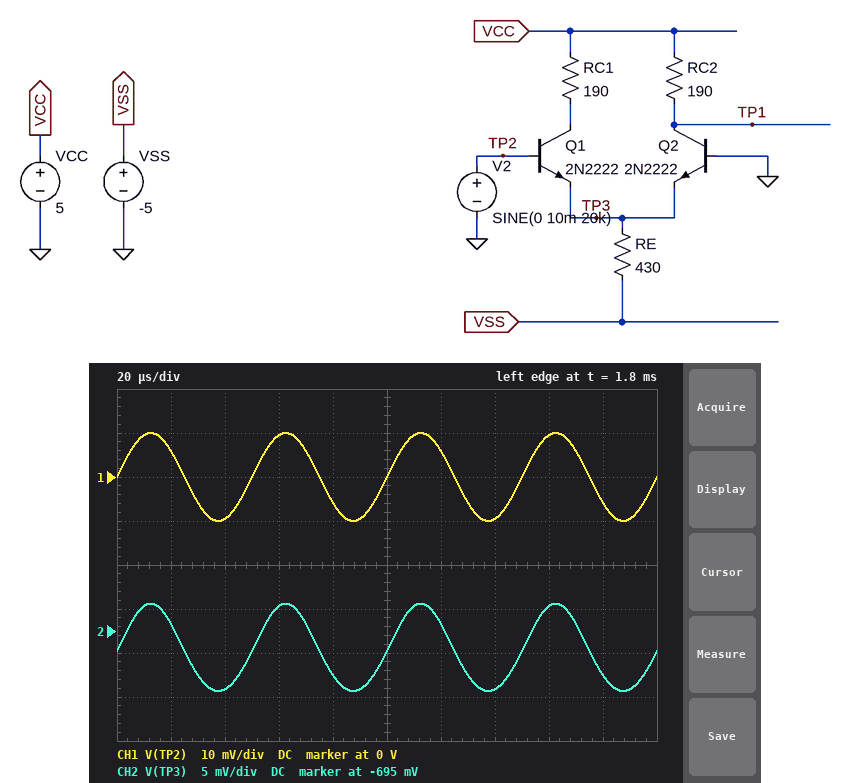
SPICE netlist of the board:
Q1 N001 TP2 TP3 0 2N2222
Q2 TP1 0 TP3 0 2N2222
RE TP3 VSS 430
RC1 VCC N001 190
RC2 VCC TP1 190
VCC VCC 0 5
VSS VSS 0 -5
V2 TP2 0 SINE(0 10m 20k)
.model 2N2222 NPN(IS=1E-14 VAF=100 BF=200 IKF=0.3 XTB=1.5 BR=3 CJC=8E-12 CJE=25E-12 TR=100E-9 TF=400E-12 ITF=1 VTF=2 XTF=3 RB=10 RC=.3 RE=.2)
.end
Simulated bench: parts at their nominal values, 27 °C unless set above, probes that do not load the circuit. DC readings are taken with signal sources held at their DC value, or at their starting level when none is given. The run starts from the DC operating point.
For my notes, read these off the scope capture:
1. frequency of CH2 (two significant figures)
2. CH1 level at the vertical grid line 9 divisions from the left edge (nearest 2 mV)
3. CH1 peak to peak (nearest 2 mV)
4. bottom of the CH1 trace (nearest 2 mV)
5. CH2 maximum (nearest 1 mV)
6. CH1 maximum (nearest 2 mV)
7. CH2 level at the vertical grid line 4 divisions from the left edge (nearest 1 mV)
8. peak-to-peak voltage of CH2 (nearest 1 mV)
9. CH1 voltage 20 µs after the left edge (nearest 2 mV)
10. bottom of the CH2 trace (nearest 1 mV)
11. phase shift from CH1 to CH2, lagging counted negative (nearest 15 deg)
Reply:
20 kHz
-6 mV
20 mV
-10 mV
-692 mV
10 mV
-700 mV
10 mV
6 mV
-702 mV
0 deg
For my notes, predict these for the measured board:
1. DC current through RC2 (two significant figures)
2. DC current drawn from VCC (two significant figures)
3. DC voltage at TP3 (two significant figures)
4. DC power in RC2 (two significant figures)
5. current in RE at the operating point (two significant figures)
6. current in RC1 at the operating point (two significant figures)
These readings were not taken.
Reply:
5.0 mA
10 mA
-700 mV
4.7 mW
10 mA
5.0 mA
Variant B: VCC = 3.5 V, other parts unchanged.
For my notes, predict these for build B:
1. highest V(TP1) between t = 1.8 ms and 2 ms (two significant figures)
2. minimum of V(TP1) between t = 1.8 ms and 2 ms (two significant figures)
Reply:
2.7 V
2.4 V
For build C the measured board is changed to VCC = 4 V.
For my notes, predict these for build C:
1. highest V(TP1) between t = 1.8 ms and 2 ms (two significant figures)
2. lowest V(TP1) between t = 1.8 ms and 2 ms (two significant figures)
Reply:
3.2 V
2.9 V
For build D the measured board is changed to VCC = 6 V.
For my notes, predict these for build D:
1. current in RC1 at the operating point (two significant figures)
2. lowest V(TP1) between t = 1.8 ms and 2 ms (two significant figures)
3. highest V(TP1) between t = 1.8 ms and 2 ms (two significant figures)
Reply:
5.0 mA
4.9 V
5.2 V
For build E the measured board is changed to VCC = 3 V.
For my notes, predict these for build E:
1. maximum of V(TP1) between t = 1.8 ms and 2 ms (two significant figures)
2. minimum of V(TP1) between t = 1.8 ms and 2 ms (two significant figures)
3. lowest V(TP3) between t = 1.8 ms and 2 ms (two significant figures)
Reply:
2.2 V
1.9 V
-700 mV
